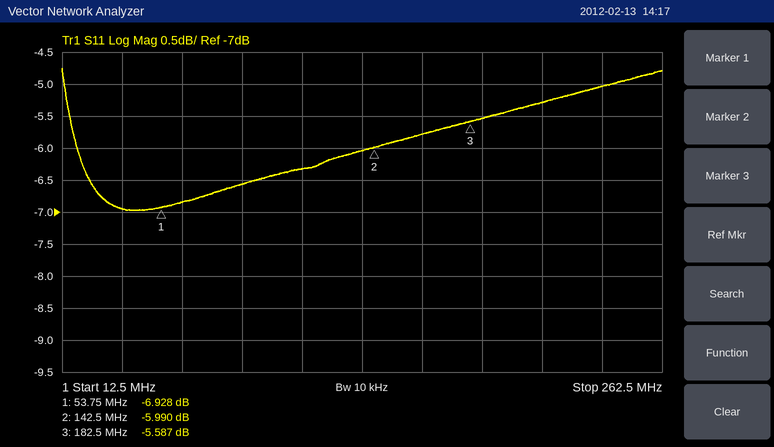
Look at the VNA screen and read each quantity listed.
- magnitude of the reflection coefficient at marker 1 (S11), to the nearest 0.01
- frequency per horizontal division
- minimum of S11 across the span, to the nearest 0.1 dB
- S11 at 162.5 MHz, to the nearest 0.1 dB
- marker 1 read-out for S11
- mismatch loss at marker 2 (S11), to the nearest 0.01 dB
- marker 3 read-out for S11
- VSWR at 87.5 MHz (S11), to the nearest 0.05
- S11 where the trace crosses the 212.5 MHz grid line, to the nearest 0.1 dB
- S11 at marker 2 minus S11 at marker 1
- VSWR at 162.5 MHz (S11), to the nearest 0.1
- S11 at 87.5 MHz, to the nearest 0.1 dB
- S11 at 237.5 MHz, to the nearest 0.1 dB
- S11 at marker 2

0.45
25 MHz
-7.0 dB
-5.8 dB
-6.928 dB
1.26 dB
-5.587 dB
2.75
-5.3 dB
0.938 dB
3.1
-6.6 dB
-5.0 dB
-5.990 dB
